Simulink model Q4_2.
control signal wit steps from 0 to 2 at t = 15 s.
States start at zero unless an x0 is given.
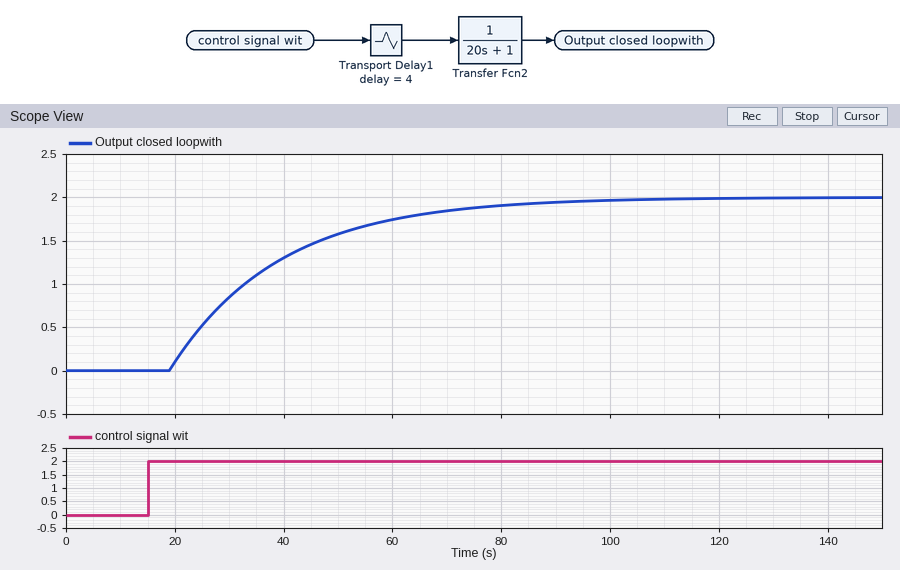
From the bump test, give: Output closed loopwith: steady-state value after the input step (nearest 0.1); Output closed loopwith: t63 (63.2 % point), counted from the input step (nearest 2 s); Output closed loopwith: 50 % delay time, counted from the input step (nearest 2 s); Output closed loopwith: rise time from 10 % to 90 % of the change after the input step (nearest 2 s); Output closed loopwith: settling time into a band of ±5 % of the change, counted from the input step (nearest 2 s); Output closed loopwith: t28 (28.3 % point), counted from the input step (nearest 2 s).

2.0
24 s
18 s
44 s
64 s
10 s
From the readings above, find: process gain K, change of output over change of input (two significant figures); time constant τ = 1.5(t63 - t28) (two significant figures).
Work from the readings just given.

1.0
21 s
